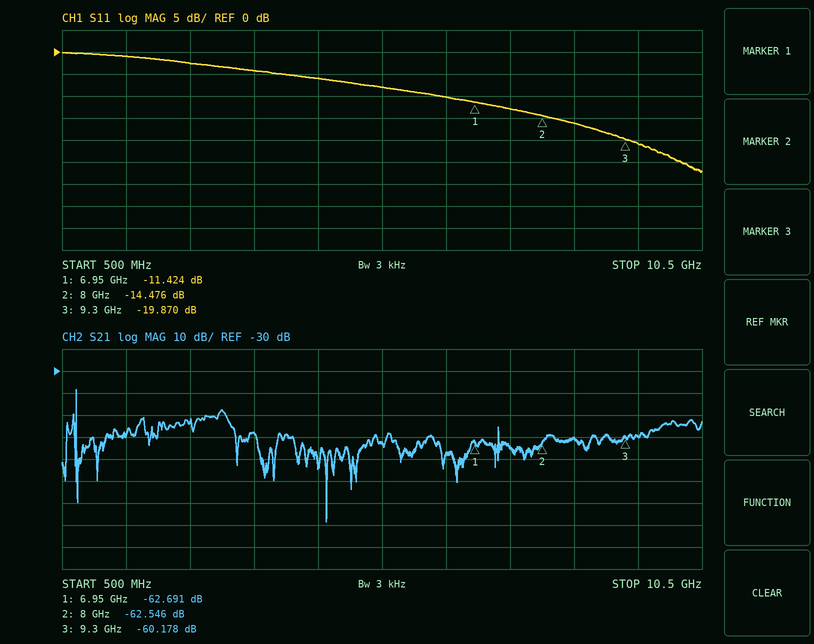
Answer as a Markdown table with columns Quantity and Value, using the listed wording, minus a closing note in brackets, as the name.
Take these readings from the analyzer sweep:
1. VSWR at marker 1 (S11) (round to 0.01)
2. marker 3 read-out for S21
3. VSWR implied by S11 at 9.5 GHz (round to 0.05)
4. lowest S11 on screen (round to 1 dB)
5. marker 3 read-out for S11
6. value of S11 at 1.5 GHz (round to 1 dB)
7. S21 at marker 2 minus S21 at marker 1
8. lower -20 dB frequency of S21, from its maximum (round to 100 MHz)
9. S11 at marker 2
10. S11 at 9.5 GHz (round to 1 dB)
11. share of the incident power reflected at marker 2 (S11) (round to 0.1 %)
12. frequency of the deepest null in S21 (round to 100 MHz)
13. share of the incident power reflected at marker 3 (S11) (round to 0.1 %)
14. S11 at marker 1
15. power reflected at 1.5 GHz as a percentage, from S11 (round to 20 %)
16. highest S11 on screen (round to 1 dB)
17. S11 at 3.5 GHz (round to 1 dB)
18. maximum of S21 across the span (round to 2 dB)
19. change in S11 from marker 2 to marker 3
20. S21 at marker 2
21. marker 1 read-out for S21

| Quantity | Value |
|---|---|
| VSWR at marker 1 (S11) | 1.73 |
| marker 3 read-out for S21 | -60.178 dB |
| VSWR implied by S11 at 9.5 GHz | 1.20 |
| lowest S11 on screen | -27 dB |
| marker 3 read-out for S11 | -19.870 dB |
| value of S11 at 1.5 GHz | -1 dB |
| S21 at marker 2 minus S21 at marker 1 | 0.145 dB |
| lower -20 dB frequency of S21, from its maximum | 700 MHz |
| S11 at marker 2 | -14.476 dB |
| S11 at 9.5 GHz | -21 dB |
| share of the incident power reflected at marker 2 (S11) | 3.6 % |
| frequency of the deepest null in S21 | 4.6 GHz |
| share of the incident power reflected at marker 3 (S11) | 1.0 % |
| S11 at marker 1 | -11.424 dB |
| power reflected at 1.5 GHz as a percentage, from S11 | 80 % |
| highest S11 on screen | 0 dB |
| S11 at 3.5 GHz | -4 dB |
| maximum of S21 across the span | -38 dB |
| change in S11 from marker 2 to marker 3 | -5.394 dB |
| S21 at marker 2 | -62.546 dB |
| marker 1 read-out for S21 | -62.691 dB |
